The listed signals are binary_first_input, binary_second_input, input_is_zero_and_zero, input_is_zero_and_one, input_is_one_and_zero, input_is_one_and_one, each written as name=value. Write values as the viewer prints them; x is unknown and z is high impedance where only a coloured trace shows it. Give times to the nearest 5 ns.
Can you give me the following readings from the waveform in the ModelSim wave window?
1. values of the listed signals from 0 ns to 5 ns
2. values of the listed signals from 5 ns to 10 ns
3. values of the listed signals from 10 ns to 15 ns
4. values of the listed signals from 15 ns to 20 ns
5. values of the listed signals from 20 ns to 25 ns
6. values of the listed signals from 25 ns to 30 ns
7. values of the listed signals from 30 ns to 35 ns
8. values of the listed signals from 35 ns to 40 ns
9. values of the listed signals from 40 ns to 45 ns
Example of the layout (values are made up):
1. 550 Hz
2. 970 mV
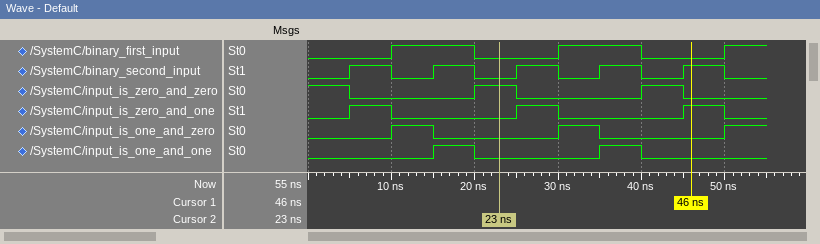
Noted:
1. binary_first_input=0, binary_second_input=0, input_is_zero_and_zero=1, input_is_zero_and_one=0, input_is_one_and_zero=0, input_is_one_and_one=0
2. binary_first_input=0, binary_second_input=1, input_is_zero_and_zero=0, input_is_zero_and_one=1, input_is_one_and_zero=0, input_is_one_and_one=0
3. binary_first_input=1, binary_second_input=0, input_is_zero_and_zero=0, input_is_zero_and_one=0, input_is_one_and_zero=1, input_is_one_and_one=0
4. binary_first_input=1, binary_second_input=1, input_is_zero_and_zero=0, input_is_zero_and_one=0, input_is_one_and_zero=0, input_is_one_and_one=1
5. binary_first_input=0, binary_second_input=0, input_is_zero_and_zero=1, input_is_zero_and_one=0, input_is_one_and_zero=0, input_is_one_and_one=0
6. binary_first_input=0, binary_second_input=1, input_is_zero_and_zero=0, input_is_zero_and_one=1, input_is_one_and_zero=0, input_is_one_and_one=0
7. binary_first_input=1, binary_second_input=0, input_is_zero_and_zero=0, input_is_zero_and_one=0, input_is_one_and_zero=1, input_is_one_and_one=0
8. binary_first_input=1, binary_second_input=1, input_is_zero_and_zero=0, input_is_zero_and_one=0, input_is_one_and_zero=0, input_is_one_and_one=1
9. binary_first_input=0, binary_second_input=0, input_is_zero_and_zero=1, input_is_zero_and_one=0, input_is_one_and_zero=0, input_is_one_and_one=0
